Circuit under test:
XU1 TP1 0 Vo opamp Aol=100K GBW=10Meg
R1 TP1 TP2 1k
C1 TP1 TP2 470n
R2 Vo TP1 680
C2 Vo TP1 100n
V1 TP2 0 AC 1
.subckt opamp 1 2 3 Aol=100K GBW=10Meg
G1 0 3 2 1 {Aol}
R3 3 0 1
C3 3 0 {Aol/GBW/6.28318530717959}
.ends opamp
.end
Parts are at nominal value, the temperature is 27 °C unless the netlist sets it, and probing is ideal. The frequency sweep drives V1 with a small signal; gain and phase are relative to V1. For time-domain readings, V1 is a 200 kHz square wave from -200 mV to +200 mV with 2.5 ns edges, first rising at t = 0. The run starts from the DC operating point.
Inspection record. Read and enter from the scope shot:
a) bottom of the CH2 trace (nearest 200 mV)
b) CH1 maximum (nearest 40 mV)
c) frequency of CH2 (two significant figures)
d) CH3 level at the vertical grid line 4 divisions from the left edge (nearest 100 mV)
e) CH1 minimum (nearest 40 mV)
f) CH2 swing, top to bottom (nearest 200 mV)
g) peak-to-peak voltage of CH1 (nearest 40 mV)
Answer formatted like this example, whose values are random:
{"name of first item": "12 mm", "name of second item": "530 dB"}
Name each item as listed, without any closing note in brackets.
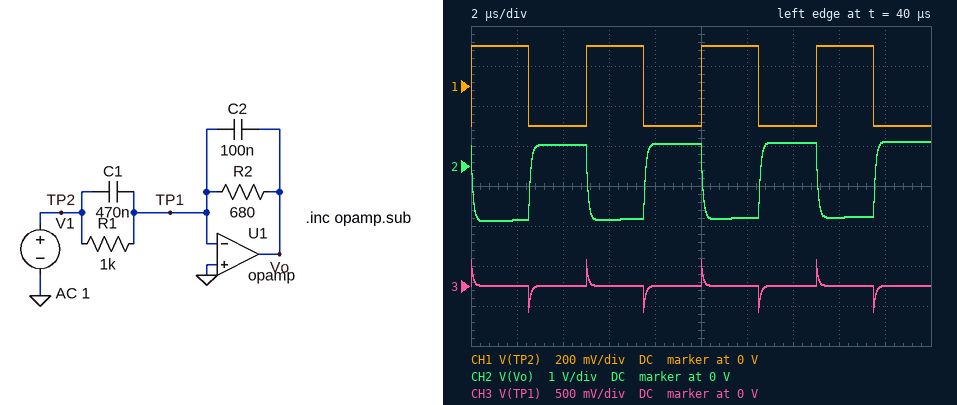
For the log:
{"bottom of the CH2 trace": "-1.4 V", "CH1 maximum": "200 mV", "frequency of CH2": "200 kHz", "CH3 level at the vertical grid line 4 divisions from the left edge": "0 V", "CH1 minimum": "-200 mV", "CH2 swing, top to bottom": "2.0 V", "peak-to-peak voltage of CH1": "400 mV"}
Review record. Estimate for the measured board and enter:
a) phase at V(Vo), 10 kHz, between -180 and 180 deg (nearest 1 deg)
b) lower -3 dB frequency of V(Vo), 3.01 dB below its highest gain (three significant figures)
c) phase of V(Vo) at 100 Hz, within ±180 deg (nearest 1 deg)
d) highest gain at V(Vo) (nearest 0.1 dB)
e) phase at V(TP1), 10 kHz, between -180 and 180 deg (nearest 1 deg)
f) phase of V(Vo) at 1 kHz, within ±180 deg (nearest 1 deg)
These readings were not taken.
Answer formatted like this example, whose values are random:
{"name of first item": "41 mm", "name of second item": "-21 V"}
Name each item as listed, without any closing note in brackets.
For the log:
{"phase at V(Vo), 10 kHz, between -180 and 180 deg": "-169 deg", "lower -3 dB frequency of V(Vo), 3.01 dB below its highest gain": "2.29 kHz", "phase of V(Vo) at 100 Hz, within ±180 deg": "-166 deg", "highest gain at V(Vo)": "13.4 dB", "phase at V(TP1), 10 kHz, between -180 and 180 deg": "100 deg", "phase of V(Vo) at 1 kHz, within ±180 deg": "-132 deg"}
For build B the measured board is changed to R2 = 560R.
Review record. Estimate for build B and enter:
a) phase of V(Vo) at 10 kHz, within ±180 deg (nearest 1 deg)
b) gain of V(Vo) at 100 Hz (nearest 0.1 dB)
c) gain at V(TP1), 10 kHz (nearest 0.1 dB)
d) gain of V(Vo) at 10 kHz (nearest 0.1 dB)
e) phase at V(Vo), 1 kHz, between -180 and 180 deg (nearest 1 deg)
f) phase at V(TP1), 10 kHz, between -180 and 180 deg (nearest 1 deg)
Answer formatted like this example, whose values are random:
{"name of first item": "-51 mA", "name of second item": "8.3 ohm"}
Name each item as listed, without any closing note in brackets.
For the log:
{"phase of V(Vo) at 10 kHz, within ±180 deg": "-166 deg", "gain of V(Vo) at 100 Hz": "-4.7 dB", "gain at V(TP1), 10 kHz": "-46.9 dB", "gain of V(Vo) at 10 kHz": "13.1 dB", "phase at V(Vo), 1 kHz, between -180 and 180 deg": "-128 deg", "phase at V(TP1), 10 kHz, between -180 and 180 deg": "103 deg"}
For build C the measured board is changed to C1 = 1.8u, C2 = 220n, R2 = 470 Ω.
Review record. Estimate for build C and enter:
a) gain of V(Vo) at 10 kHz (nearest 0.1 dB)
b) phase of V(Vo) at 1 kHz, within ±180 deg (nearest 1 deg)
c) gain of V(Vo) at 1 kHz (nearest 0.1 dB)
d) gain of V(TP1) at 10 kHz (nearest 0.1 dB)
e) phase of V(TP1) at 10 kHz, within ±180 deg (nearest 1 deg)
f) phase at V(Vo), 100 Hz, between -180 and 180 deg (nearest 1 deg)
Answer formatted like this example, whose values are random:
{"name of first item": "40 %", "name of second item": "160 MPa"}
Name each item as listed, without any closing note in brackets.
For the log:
{"gain of V(Vo) at 10 kHz": "18.2 dB", "phase of V(Vo) at 1 kHz, within ±180 deg": "-128 deg", "gain of V(Vo) at 1 kHz": "13.0 dB", "gain of V(TP1) at 10 kHz": "-41.8 dB", "phase of V(TP1) at 10 kHz, within ±180 deg": "97 deg", "phase at V(Vo), 100 Hz, between -180 and 180 deg": "-135 deg"}
